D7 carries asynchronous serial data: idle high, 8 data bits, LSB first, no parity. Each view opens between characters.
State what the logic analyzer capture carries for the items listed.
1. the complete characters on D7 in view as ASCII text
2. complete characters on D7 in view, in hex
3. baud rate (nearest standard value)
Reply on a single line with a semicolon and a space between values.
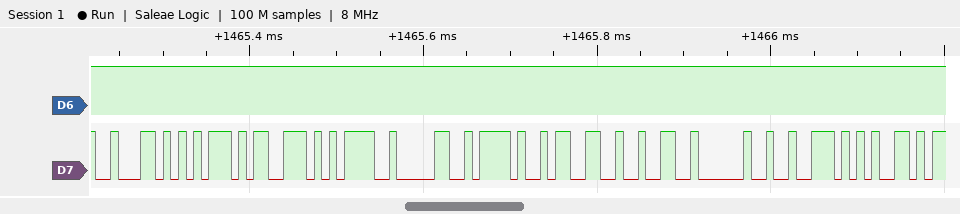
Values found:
"bus=0/32 re"; 62, 75, 73, 3D, 30, 2F, 33, 32, 20, 72, 65; 115200 baud
